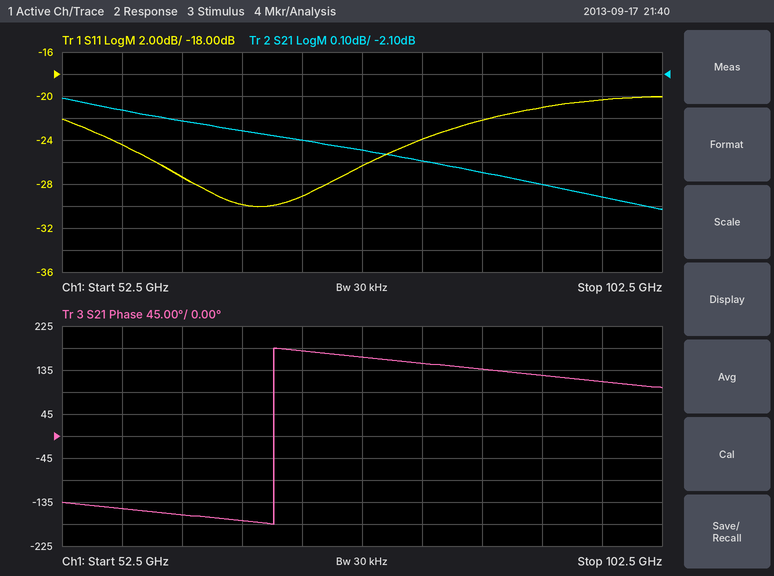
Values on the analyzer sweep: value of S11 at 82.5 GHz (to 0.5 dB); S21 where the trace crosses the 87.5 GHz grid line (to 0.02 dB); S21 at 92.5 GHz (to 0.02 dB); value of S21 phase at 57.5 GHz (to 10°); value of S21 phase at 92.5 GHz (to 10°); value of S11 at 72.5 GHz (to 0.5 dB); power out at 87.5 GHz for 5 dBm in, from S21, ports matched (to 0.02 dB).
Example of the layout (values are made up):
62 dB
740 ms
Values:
-24.0 dB
-2.54 dB
-2.60 dB
-150°
120°
-29.0 dB
2.46 dBm
